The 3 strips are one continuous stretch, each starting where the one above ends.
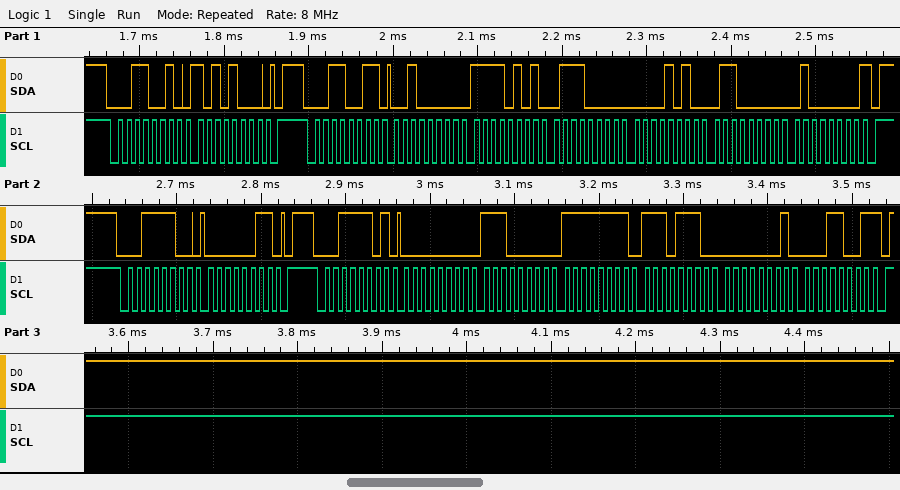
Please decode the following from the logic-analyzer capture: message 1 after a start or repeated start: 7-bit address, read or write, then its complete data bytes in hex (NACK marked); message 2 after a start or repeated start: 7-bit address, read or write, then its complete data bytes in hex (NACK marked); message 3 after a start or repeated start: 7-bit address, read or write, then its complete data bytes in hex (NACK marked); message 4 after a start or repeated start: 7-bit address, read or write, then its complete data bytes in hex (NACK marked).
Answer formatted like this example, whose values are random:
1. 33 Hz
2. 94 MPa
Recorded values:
1. 0x19 write: A8
2. 0x19 read: 20 F5 70 0A 60 40 NACK
3. 0x1E write: 03
4. 0x1E read: 00 E0 FF EE 01 19 NACK
